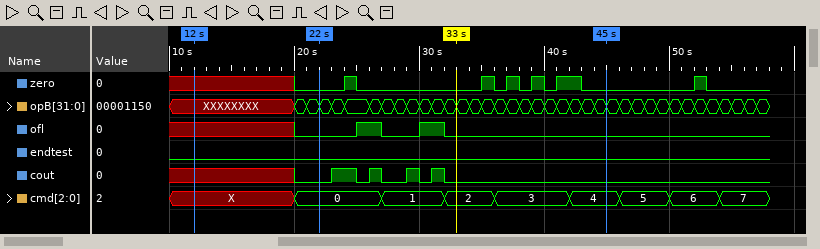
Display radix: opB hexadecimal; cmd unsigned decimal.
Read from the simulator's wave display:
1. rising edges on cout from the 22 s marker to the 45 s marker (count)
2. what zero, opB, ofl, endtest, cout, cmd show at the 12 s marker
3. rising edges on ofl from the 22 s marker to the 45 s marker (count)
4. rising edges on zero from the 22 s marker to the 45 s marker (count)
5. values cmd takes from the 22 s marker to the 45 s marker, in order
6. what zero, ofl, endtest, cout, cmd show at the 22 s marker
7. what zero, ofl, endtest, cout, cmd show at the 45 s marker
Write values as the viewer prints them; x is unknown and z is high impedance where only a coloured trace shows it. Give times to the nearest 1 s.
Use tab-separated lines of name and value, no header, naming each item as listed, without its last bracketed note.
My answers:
rising edges on cout from the 22 s marker to the 45 s marker	4
what zero, opB, ofl, endtest, cout, cmd show at the 12 s marker	zero=x, opB=XXXXXXXX, ofl=x, endtest=0, cout=x, cmd=X
rising edges on ofl from the 22 s marker to the 45 s marker	2
rising edges on zero from the 22 s marker to the 45 s marker	5
values cmd takes from the 22 s marker to the 45 s marker, in order	0, 1, 2, 3, 4
what zero, ofl, endtest, cout, cmd show at the 22 s marker	zero=0, ofl=0, endtest=0, cout=0, cmd=0
what zero, ofl, endtest, cout, cmd show at the 45 s marker	zero=0, ofl=0, endtest=0, cout=0, cmd=4
